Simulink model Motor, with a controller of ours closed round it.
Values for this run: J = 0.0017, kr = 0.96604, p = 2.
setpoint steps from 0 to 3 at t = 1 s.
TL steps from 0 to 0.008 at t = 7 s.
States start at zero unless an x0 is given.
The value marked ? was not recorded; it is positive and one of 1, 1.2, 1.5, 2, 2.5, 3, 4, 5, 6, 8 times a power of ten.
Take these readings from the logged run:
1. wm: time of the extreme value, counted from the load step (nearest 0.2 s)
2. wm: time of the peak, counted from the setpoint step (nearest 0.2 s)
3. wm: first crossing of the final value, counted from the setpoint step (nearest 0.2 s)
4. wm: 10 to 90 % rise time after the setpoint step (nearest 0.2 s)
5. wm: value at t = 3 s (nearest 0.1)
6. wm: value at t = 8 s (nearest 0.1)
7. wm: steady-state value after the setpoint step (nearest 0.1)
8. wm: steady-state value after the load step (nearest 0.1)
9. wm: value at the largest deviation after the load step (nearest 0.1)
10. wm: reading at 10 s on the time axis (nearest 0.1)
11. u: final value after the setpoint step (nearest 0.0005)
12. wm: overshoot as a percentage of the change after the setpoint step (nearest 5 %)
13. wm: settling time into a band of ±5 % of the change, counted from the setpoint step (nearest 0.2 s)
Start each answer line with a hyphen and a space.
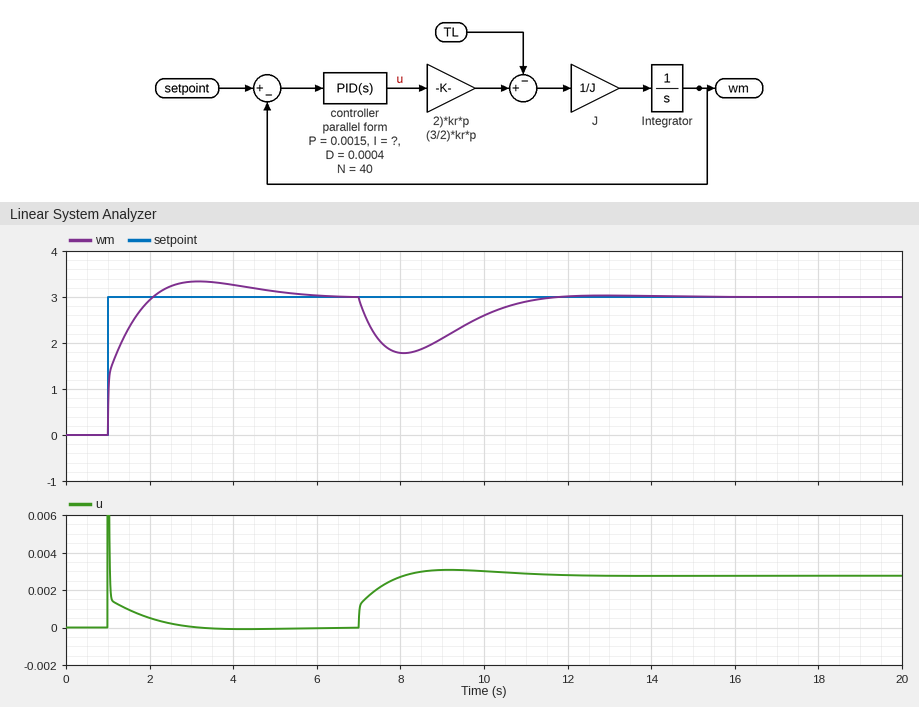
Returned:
- 1.0 s
- 2.2 s
- 1.0 s
- 0.8 s
- 3.3
- 1.8
- 3.0
- 3.0
- 1.8
- 2.6
- 0.0000
- 10 %
- 3.8 s
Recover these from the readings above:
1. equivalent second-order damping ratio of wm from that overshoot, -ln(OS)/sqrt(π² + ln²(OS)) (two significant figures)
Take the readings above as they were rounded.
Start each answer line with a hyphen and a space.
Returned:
- 0.59
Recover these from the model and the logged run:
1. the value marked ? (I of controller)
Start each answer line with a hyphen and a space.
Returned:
- 0.001
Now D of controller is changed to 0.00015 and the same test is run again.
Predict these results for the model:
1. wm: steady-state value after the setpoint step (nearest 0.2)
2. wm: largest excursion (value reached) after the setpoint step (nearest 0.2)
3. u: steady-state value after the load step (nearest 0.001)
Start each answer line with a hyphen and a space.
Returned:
- 3.0
- 3.4
- 0.003
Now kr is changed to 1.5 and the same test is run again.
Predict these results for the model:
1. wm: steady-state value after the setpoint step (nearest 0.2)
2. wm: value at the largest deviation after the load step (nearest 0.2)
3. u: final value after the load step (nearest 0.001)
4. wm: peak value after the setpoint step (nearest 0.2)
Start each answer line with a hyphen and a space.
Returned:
- 3.0
- 2.2
- 0.002
- 3.2
